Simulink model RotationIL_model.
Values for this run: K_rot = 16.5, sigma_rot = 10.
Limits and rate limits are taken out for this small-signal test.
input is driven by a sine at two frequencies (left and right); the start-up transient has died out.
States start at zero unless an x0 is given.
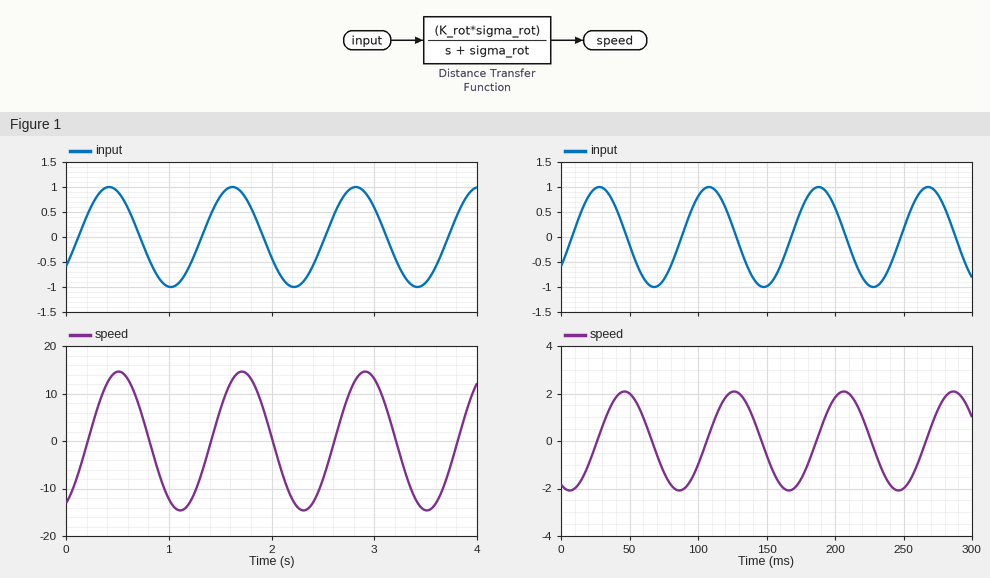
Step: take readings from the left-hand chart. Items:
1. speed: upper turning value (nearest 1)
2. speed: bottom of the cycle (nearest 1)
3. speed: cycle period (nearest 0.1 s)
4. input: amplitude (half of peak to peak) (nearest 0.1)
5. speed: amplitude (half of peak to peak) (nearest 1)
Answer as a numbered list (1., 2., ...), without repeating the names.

1. 15
2. -15
3. 1.2 s
4. 1.0
5. 15
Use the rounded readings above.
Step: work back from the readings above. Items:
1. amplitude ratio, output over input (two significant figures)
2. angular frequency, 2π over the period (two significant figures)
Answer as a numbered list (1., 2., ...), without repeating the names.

1. 15
2. 5.2 rad/s
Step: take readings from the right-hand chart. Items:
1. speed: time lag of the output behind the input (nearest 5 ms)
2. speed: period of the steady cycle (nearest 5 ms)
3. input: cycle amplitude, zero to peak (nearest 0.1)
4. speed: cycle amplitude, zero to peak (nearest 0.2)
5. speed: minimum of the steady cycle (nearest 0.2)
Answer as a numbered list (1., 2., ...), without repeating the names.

1. 20 ms
2. 80 ms
3. 1.0
4. 2.0
5. -2.0
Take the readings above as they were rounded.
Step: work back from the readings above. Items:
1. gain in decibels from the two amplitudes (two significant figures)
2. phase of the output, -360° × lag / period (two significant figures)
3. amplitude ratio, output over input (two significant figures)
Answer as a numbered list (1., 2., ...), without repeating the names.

1. 6.0 dB
2. -90°
3. 2.0
